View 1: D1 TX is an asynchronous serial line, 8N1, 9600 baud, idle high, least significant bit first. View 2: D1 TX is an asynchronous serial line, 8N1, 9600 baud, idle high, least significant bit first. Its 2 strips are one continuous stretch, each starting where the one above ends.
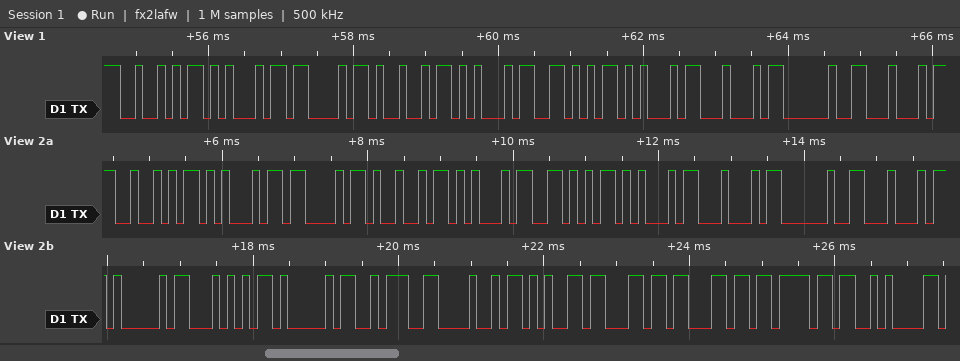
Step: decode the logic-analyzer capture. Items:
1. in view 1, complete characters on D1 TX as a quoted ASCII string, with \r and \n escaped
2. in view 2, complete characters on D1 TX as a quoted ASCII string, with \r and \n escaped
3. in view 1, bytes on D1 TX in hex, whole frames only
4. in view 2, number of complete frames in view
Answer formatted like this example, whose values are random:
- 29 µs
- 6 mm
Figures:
- "RECIEVED D"
- "RECIEVED DATA:Hello\n"
- 0x52 0x45 0x43 0x49 0x45 0x56 0x45 0x44 0x20 0x44
- 20
